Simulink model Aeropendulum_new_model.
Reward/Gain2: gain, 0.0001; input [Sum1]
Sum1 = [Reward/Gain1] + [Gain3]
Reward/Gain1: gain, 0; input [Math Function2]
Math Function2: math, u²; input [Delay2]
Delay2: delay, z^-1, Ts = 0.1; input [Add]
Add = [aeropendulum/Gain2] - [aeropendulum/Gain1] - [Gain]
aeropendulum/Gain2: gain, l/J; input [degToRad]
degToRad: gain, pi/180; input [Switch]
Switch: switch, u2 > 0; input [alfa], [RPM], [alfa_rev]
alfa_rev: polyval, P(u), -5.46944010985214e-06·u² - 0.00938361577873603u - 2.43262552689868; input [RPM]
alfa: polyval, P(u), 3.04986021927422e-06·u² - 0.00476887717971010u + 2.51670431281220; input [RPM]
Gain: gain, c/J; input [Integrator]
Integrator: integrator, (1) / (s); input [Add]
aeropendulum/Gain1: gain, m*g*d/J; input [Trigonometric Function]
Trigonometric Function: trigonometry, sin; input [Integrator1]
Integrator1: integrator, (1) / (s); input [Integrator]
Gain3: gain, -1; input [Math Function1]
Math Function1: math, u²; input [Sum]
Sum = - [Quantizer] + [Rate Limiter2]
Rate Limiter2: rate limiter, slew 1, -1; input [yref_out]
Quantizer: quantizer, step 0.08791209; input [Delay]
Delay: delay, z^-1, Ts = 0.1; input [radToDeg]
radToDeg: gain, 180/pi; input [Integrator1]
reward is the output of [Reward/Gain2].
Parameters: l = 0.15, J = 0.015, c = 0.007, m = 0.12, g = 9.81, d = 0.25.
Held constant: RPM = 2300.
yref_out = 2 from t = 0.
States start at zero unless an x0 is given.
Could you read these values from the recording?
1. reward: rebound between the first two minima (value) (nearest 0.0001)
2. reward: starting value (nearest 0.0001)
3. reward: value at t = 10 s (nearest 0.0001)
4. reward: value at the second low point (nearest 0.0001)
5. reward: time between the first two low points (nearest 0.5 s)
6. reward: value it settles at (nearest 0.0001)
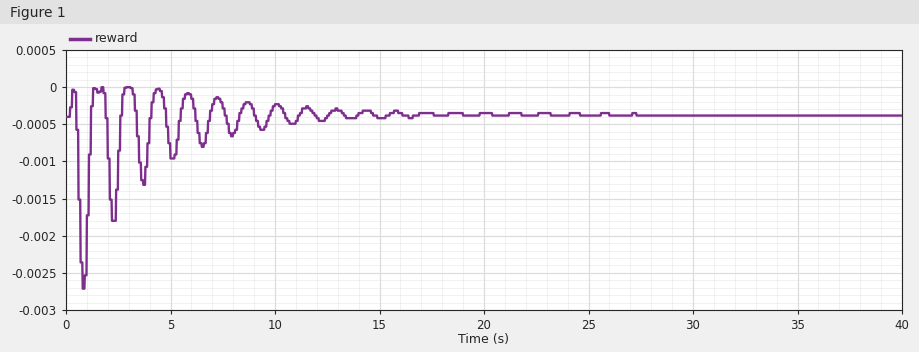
0.0000
-0.0004
-0.0002
-0.0018
1.5 s
-0.0004
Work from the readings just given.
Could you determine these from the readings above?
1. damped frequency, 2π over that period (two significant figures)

4.2 rad/s
